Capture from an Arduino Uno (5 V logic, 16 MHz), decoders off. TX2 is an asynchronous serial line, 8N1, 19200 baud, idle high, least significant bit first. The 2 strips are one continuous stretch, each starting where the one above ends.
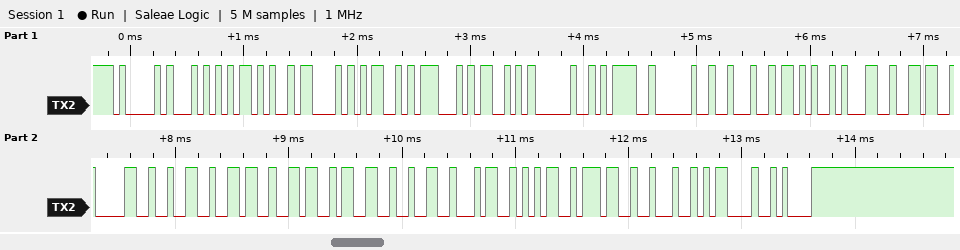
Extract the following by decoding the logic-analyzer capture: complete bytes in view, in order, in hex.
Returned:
41 54 2B 43 4D 47 53 20 3D 20 22 2B 31 36 30 32 36 36 33 32 34 35 37 22 0D 0A
